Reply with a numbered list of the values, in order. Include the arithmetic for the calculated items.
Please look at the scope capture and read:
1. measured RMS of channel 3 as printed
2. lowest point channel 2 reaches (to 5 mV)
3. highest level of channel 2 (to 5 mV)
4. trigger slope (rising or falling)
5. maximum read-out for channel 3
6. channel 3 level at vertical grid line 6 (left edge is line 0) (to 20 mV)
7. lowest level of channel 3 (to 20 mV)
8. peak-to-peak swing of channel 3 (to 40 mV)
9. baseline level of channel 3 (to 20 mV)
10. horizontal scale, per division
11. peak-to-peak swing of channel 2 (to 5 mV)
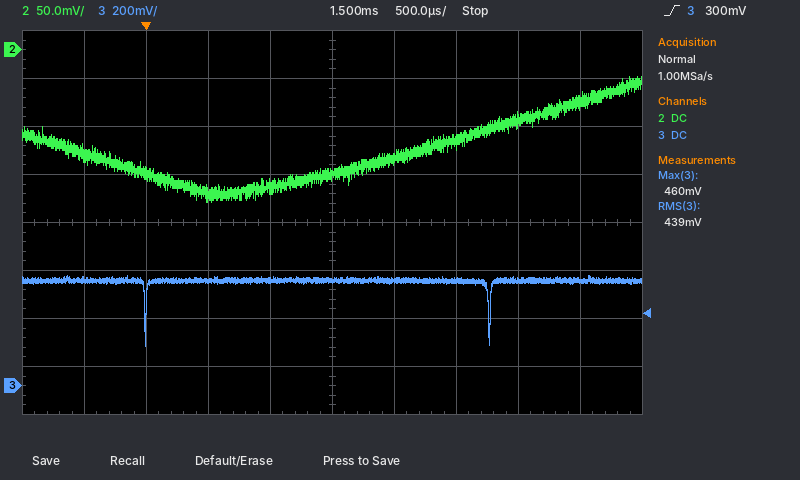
1. 439 mV
2. -160 mV
3. -30 mV
4. rising
5. 460 mV
6. 440 mV
7. 160 mV
8. 280 mV
9. 440 mV
10. 500 µs
11. -30 mV − (-160 mV) = 130 mV
